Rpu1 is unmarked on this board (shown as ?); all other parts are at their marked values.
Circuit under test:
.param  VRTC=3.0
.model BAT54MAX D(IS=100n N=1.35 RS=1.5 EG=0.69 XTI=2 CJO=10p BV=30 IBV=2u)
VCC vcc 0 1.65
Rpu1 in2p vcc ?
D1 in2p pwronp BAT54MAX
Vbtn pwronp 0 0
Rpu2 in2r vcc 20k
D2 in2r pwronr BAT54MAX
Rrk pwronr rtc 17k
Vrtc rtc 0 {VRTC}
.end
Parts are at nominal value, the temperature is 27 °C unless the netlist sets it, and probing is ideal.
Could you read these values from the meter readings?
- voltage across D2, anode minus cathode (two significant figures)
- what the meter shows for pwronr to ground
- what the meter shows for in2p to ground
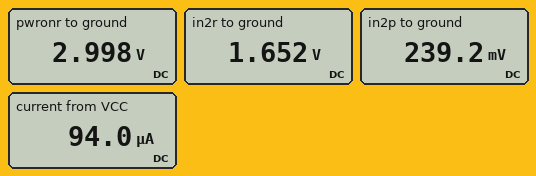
-1.3 V
2.998 V
239.2 mV
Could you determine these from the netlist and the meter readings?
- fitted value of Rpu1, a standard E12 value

15 kΩ
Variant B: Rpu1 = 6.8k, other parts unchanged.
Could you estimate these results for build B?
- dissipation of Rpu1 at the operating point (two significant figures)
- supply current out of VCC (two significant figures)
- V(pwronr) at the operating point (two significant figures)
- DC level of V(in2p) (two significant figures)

280 µW
200 µA
3.0 V
270 mV
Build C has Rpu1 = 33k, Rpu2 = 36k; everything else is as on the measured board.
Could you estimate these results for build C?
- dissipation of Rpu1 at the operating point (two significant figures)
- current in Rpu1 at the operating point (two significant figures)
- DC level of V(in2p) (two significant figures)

63 µW
44 µA
210 mV
